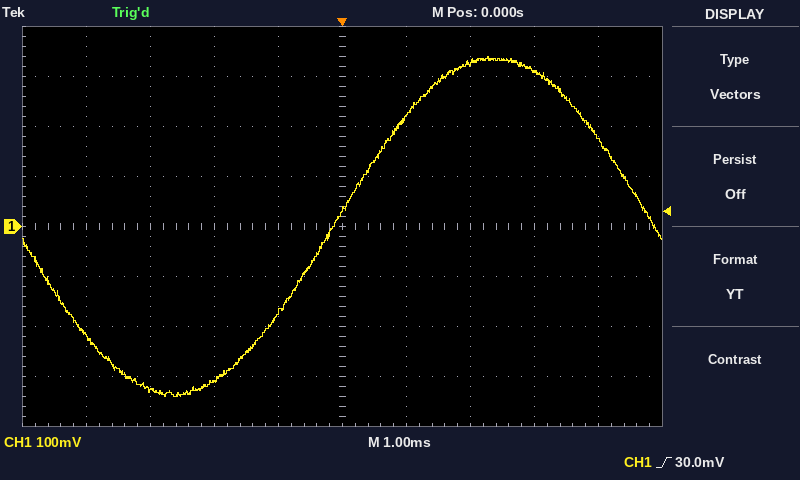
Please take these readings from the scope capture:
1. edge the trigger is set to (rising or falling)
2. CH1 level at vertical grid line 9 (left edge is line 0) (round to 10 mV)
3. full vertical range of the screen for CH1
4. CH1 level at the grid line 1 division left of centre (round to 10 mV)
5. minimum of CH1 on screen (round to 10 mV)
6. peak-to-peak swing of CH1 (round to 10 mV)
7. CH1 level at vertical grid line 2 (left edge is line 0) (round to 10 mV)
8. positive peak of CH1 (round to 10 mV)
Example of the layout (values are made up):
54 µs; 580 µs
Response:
rising; 180 mV; 800 mV; -170 mV; -340 mV; 680 mV; -330 mV; 340 mV
